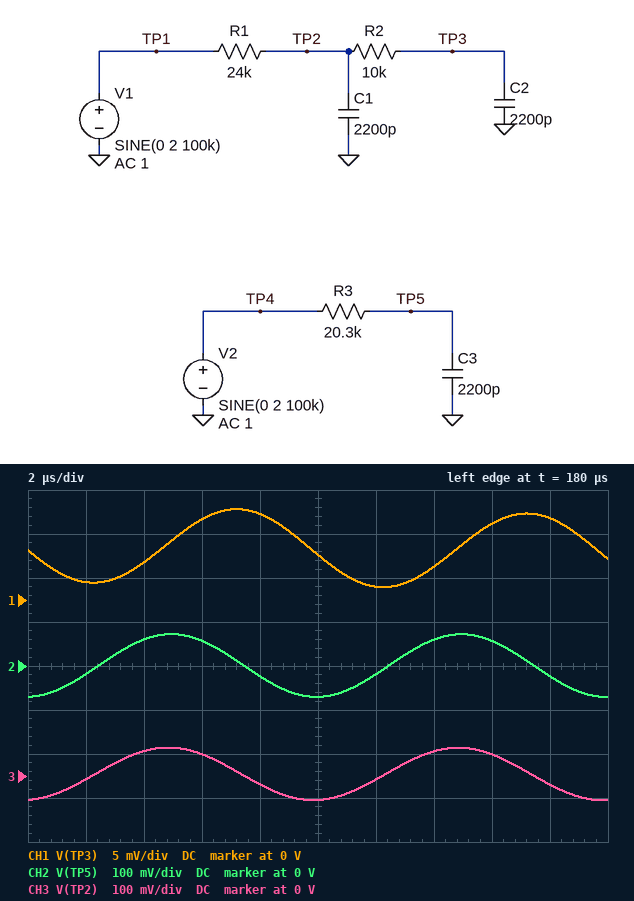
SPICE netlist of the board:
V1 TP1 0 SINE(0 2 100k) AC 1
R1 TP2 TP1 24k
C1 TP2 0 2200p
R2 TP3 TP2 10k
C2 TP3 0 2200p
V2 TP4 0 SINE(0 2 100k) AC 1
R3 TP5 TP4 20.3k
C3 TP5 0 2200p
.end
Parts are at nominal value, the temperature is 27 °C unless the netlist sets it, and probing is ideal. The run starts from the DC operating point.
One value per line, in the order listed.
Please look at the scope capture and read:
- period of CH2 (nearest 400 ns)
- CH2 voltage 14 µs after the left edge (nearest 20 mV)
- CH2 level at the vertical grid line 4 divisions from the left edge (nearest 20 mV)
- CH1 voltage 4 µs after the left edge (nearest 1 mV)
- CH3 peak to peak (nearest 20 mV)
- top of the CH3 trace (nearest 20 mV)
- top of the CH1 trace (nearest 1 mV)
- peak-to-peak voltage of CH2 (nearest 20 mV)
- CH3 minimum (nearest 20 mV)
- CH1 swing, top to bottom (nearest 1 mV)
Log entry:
10.0 µs
60 mV
-20 mV
4 mV
120 mV
60 mV
10 mV
140 mV
-60 mV
9 mV
